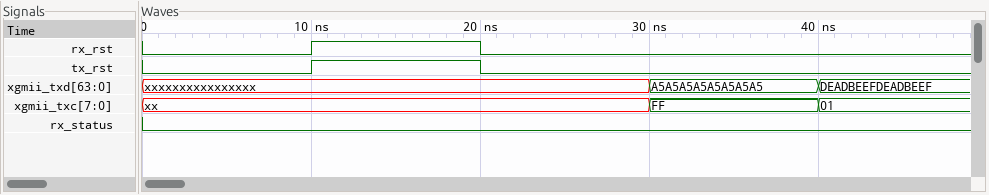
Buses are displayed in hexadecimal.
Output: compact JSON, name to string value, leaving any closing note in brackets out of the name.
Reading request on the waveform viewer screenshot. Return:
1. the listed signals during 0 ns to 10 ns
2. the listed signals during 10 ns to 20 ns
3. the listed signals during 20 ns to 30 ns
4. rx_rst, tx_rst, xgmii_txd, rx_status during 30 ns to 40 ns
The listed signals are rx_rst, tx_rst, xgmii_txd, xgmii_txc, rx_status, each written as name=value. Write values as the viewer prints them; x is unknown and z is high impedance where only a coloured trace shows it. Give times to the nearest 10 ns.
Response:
{"the listed signals during 0 ns to 10 ns": "rx_rst=0, tx_rst=0, xgmii_txd=xxxxxxxxxxxxxxxx, xgmii_txc=xx, rx_status=0", "the listed signals during 10 ns to 20 ns": "rx_rst=1, tx_rst=1, xgmii_txd=xxxxxxxxxxxxxxxx, xgmii_txc=xx, rx_status=0", "the listed signals during 20 ns to 30 ns": "rx_rst=0, tx_rst=0, xgmii_txd=xxxxxxxxxxxxxxxx, xgmii_txc=xx, rx_status=0", "rx_rst, tx_rst, xgmii_txd, rx_status during 30 ns to 40 ns": "rx_rst=0, tx_rst=0, xgmii_txd=A5A5A5A5A5A5A5A5, rx_status=0"}
